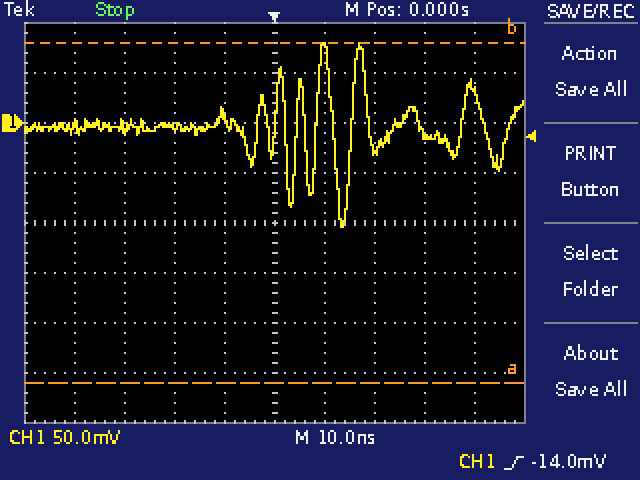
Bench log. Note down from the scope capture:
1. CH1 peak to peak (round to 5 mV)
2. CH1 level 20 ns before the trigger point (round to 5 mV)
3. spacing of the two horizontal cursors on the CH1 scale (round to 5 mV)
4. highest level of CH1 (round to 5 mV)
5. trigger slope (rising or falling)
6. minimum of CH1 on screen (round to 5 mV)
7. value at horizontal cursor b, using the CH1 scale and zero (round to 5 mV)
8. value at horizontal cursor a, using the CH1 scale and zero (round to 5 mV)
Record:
185 mV
-5 mV
340 mV
80 mV
rising
-105 mV
80 mV
-260 mV
